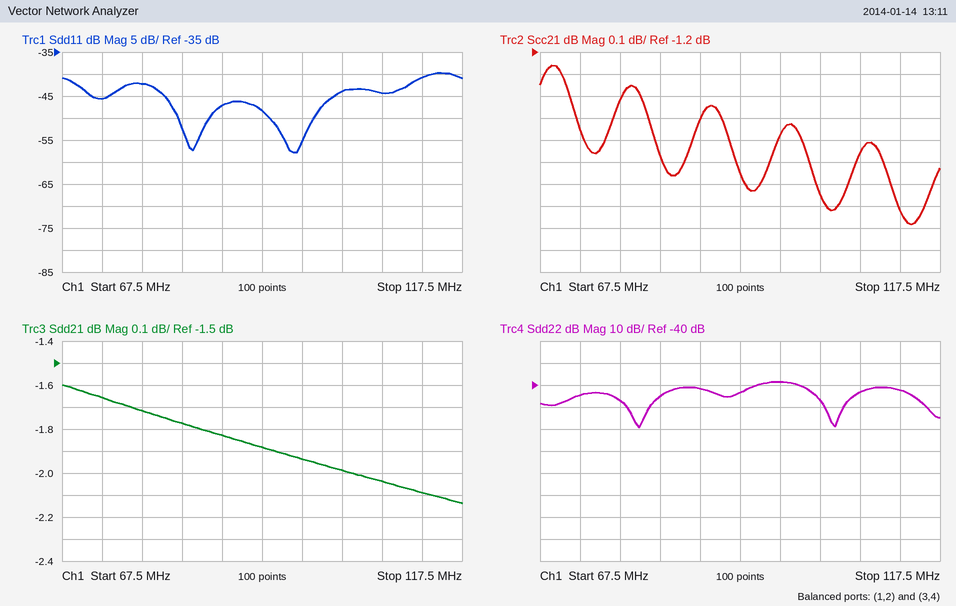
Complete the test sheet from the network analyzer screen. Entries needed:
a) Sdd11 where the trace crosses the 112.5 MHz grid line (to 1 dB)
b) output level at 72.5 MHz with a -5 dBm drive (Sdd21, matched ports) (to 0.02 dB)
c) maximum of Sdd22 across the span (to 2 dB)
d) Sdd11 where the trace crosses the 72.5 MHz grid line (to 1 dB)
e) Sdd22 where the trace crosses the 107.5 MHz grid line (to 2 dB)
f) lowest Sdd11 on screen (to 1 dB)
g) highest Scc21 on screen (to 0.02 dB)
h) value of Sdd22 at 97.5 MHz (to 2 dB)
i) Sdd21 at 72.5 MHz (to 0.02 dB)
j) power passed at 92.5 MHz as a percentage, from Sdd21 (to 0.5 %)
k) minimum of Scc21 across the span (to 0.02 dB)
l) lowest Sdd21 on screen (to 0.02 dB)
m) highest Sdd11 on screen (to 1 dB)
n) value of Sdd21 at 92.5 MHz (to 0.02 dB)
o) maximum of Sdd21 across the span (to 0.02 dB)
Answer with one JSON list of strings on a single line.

["-41 dB", "-6.66 dBm", "-38 dB", "-46 dB", "-44 dB", "-58 dB", "-1.26 dB", "-38 dB", "-1.66 dB", "65.0 %", "-1.98 dB", "-2.14 dB", "-40 dB", "-1.88 dB", "-1.60 dB"]
